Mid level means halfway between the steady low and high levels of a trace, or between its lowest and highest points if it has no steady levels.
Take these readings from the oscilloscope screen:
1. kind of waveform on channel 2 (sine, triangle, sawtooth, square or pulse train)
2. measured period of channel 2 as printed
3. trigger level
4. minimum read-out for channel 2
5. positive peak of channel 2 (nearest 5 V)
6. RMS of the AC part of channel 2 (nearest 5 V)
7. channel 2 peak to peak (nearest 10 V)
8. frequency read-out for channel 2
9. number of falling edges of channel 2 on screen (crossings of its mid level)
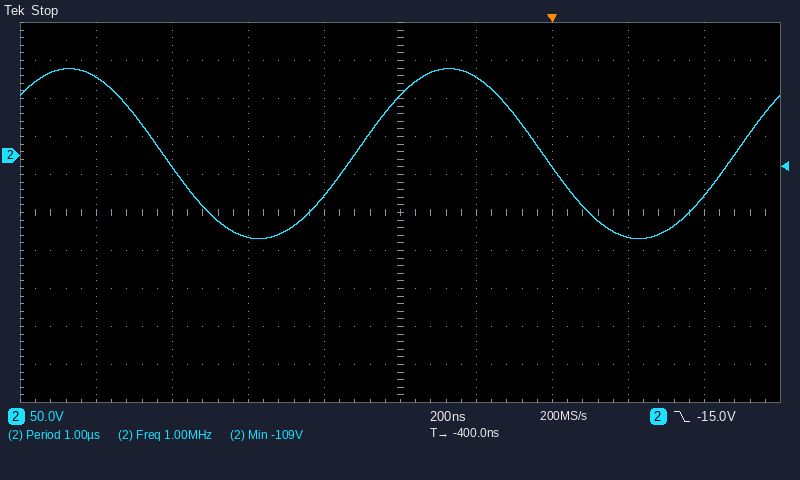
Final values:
sine
1.00 µs
-15.0 V
-109 V
115 V
80 V
220 V
1.00 MHz
2
